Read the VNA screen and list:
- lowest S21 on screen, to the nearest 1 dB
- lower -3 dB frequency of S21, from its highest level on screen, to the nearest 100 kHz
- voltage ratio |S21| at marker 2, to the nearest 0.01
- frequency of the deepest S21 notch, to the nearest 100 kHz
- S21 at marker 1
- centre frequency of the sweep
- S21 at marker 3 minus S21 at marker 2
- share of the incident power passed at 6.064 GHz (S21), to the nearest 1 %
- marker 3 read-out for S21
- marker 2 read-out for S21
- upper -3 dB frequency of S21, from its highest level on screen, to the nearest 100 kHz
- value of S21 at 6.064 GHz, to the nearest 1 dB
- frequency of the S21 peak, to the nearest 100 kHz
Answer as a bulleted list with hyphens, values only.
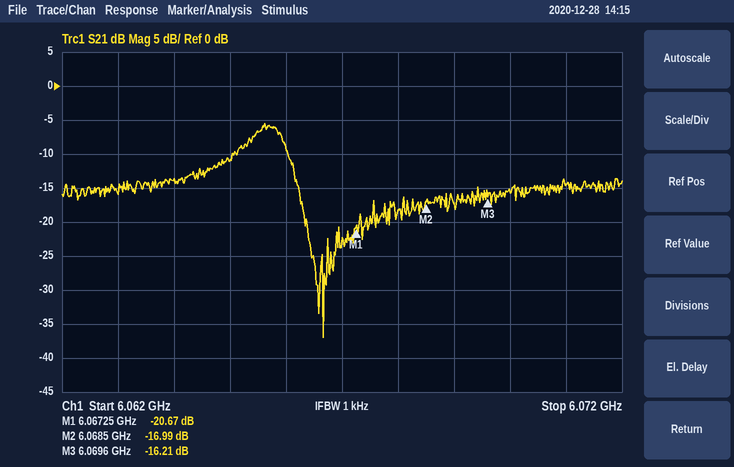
- -37 dB
- 6.0653 GHz
- 0.14
- 6.0667 GHz
- -20.67 dB
- 6.067 GHz
- 0.78 dB
- 4 %
- -16.21 dB
- -16.99 dB
- 6.0660 GHz
- -14 dB
- 6.0656 GHz
